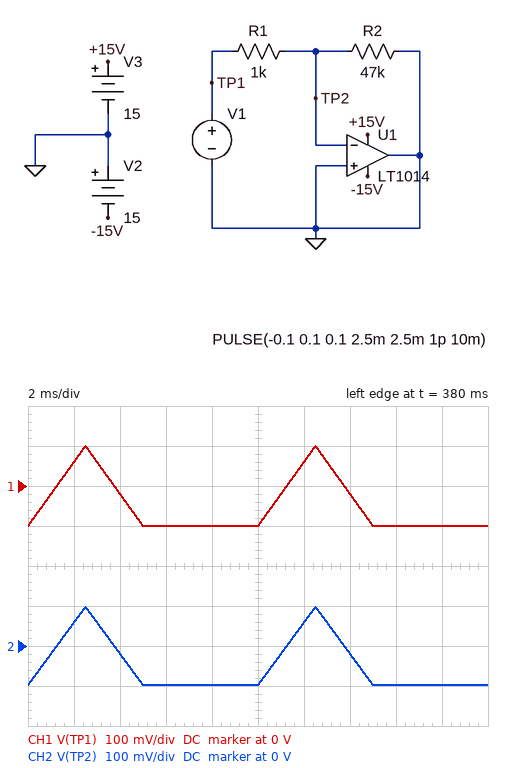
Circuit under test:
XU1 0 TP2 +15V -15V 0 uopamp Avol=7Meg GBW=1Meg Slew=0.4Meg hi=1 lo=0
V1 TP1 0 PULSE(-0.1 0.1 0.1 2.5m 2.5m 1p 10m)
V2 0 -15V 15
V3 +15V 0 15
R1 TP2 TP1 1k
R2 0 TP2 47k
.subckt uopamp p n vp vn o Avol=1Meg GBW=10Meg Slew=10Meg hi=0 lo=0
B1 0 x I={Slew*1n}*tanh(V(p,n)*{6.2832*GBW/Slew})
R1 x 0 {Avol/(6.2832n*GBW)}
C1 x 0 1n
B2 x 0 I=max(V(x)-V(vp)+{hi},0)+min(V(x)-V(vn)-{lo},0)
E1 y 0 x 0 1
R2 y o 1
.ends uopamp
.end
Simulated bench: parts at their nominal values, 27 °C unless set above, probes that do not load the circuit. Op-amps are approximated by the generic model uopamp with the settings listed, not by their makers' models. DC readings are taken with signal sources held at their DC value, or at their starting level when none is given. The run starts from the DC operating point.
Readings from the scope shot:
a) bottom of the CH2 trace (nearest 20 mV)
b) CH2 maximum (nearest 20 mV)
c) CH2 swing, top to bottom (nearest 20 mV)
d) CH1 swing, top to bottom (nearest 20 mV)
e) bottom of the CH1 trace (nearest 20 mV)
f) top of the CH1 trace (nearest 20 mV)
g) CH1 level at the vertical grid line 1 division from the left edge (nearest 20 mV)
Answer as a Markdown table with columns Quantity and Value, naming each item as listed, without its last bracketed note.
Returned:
| Quantity | Value |
|---|---|
| bottom of the CH2 trace | -100 mV |
| CH2 maximum | 100 mV |
| CH2 swing, top to bottom | 200 mV |
| CH1 swing, top to bottom | 200 mV |
| bottom of the CH1 trace | -100 mV |
| top of the CH1 trace | 100 mV |
| CH1 level at the vertical grid line 1 division from the left edge | 60 mV |
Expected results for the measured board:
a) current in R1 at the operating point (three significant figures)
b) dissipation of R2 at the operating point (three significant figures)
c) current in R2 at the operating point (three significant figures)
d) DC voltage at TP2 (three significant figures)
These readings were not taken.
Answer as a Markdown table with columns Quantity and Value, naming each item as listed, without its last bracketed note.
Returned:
| Quantity | Value |
|---|---|
| current in R1 at the operating point | 2.08 µA |
| dissipation of R2 at the operating point | 204 nW |
| current in R2 at the operating point | 2.08 µA |
| DC voltage at TP2 | -97.9 mV |
